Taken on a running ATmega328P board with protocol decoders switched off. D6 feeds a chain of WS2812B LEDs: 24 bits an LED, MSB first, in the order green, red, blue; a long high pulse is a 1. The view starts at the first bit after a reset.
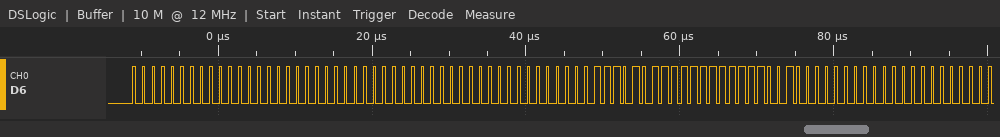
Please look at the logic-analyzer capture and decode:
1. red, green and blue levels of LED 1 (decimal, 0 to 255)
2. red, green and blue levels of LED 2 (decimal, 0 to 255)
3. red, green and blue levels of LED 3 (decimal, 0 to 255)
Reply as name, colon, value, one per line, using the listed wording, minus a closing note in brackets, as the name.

red, green and blue levels of LED 1: 0, 0, 0
red, green and blue levels of LED 2: 0, 0, 0
red, green and blue levels of LED 3: 255, 235, 200
